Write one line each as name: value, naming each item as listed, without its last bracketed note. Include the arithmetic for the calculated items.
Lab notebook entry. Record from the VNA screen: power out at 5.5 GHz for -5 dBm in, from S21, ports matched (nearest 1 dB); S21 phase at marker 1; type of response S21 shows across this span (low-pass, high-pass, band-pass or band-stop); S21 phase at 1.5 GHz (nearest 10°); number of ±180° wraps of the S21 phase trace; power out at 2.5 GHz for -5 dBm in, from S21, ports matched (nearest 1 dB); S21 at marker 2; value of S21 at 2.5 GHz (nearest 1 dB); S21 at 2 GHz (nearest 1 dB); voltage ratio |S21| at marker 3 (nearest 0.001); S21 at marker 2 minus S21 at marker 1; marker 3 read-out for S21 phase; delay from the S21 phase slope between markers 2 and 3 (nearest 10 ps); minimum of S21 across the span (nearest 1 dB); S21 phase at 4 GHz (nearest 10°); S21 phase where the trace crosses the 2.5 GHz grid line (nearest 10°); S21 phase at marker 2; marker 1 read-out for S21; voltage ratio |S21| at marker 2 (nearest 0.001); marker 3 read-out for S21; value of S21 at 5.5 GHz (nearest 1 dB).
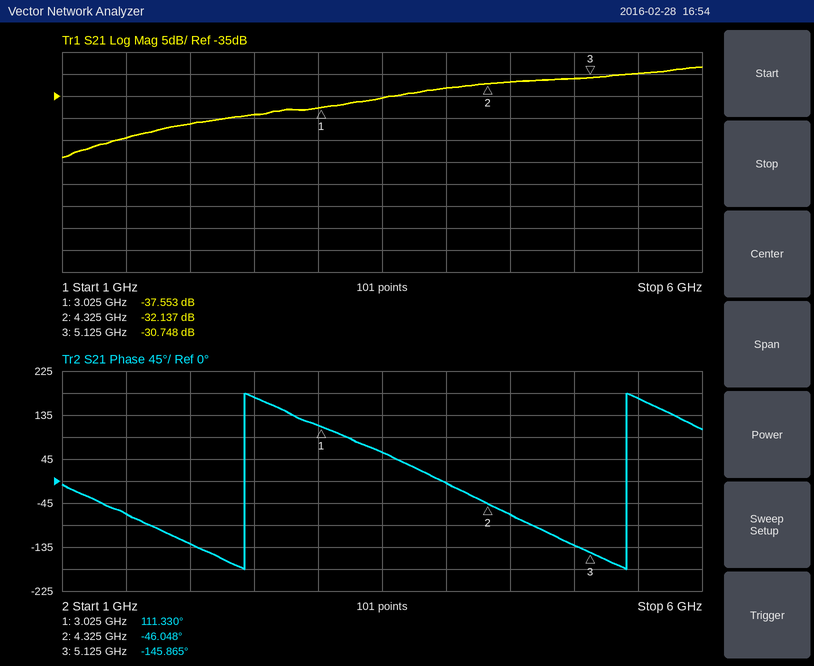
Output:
power out at 5.5 GHz for -5 dBm in, from S21, ports matched: -5 dBm + (-30 dB) = -35 dBm
S21 phase at marker 1: 111.330°
type of response S21 shows across this span: high-pass
S21 phase at 1.5 GHz: -70°
number of ±180° wraps of the S21 phase trace: 2
power out at 2.5 GHz for -5 dBm in, from S21, ports matched: -5 dBm + (-39 dB) = -44 dBm
S21 at marker 2: -32.137 dB
value of S21 at 2.5 GHz: -39 dB
S21 at 2 GHz: -41 dB
voltage ratio |S21| at marker 3: 10^(-30.748/20) ≈ 0.029
S21 at marker 2 minus S21 at marker 1: -32.137 − (-37.553) = 5.416 dB
marker 3 read-out for S21 phase: -145.865°
delay from the S21 phase slope between markers 2 and 3: −(-145.865° − (-46.048°))/(360° × 800 MHz) ≈ 347 ps, so 350 ps to the nearest 10 ps
minimum of S21 across the span: -49 dB
S21 phase at 4 GHz: 0°
S21 phase where the trace crosses the 2.5 GHz grid line: 170°
S21 phase at marker 2: -46.048°
marker 1 read-out for S21: -37.553 dB
voltage ratio |S21| at marker 2: 10^(-32.137/20) ≈ 0.025
marker 3 read-out for S21: -30.748 dB
value of S21 at 5.5 GHz: -30 dB
